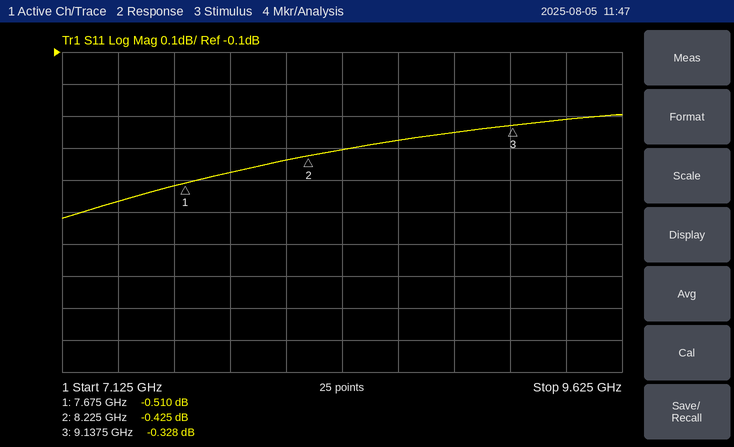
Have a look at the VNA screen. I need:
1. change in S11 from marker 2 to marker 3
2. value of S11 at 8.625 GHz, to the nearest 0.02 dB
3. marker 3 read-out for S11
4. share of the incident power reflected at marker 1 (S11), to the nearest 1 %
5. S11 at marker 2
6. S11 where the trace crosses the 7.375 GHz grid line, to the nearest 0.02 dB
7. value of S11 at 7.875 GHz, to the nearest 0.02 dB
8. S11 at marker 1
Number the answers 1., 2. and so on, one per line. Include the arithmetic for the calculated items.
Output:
1. -0.328 − (-0.425) = 0.097 dB
2. -0.38 dB
3. -0.328 dB
4. 10^(-0.51/10) ≈ 89 %
5. -0.425 dB
6. -0.56 dB
7. -0.48 dB
8. -0.510 dB
